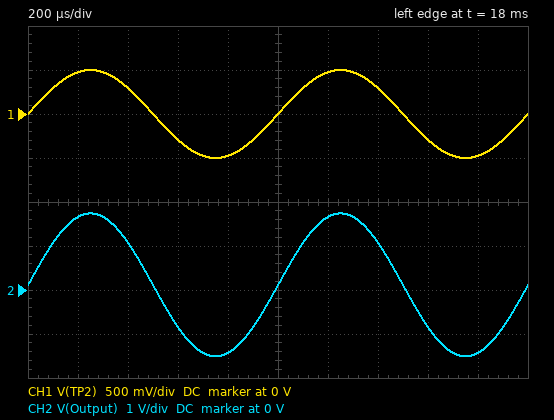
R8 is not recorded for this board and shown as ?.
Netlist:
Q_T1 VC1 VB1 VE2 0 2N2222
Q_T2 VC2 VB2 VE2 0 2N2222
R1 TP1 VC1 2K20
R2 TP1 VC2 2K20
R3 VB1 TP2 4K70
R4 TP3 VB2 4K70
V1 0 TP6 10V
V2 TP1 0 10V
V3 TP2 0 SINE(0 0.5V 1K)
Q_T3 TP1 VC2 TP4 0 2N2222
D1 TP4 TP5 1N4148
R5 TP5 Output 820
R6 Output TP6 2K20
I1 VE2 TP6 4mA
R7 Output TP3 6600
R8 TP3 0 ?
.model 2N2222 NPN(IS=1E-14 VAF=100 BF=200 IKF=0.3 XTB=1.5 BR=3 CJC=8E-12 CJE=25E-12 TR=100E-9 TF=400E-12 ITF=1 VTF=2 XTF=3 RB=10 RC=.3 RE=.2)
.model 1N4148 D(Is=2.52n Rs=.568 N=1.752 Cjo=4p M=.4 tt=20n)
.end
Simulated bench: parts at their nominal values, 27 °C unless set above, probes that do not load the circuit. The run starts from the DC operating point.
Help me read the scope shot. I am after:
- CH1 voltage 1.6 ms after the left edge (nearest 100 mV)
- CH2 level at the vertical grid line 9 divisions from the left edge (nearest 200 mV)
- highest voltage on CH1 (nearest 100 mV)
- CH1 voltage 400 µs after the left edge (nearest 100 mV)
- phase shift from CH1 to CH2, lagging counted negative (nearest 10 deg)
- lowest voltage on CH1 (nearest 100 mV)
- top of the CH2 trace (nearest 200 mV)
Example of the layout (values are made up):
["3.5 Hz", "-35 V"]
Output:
["-300 mV", "-1.4 V", "500 mV", "300 mV", "0 deg", "-500 mV", "1.8 V"]
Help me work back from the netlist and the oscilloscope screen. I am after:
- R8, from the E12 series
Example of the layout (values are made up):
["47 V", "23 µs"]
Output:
["2.2 kΩ"]
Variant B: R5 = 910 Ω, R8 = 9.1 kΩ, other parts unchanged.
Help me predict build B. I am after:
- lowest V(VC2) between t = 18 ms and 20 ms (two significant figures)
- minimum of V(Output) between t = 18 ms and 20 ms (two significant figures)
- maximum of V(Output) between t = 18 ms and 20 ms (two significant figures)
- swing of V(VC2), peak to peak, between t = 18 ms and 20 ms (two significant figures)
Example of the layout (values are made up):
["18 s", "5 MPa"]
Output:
["4.4 V", "-720 mV", "840 mV", "2.3 V"]
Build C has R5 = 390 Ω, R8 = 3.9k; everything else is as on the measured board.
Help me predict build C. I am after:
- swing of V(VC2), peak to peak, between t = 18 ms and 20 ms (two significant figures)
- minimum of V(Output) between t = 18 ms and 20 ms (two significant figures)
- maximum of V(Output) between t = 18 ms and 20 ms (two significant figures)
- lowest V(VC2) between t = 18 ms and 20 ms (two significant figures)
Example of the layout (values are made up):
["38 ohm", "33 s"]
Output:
["2.9 V", "-870 mV", "1.5 V", "2.1 V"]
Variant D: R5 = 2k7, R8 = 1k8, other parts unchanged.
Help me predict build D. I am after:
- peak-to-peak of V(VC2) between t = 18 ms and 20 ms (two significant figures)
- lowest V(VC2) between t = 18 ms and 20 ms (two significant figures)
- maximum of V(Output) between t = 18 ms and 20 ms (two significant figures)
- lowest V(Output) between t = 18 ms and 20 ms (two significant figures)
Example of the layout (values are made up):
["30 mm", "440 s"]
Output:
["2.8 V", "7.1 V", "-1.4 V", "-2.5 V"]
